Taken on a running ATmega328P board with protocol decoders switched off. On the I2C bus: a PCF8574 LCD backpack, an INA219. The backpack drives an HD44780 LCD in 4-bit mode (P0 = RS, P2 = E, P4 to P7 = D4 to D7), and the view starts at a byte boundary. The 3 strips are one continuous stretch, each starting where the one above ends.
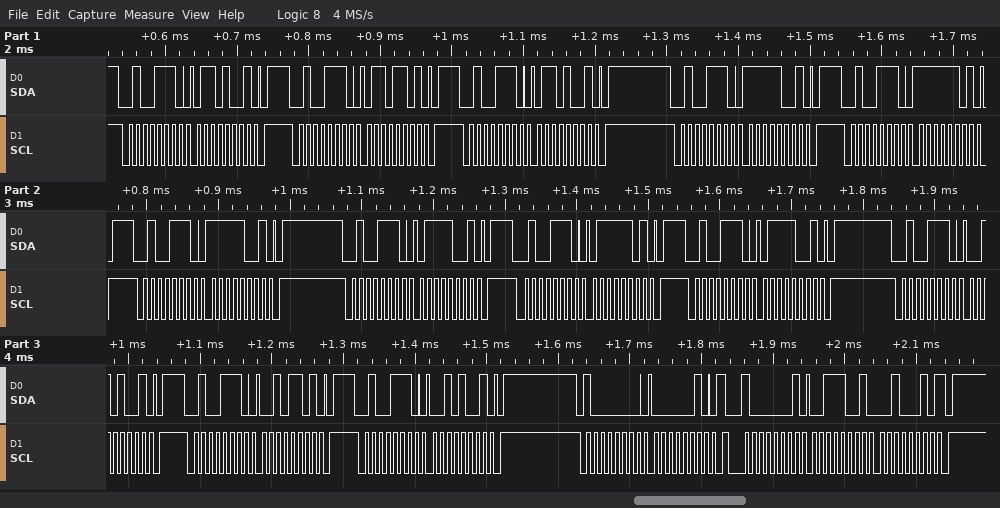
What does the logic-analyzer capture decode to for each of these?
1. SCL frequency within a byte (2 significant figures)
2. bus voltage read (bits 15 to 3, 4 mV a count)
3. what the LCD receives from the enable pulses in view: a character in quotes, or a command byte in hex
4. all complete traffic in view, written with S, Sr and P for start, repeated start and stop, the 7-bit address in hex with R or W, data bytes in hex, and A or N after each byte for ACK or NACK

100 kHz
7.312 V
'o' 'r'
S 27W A 69 A P S 27W A 6D A P S 27W A 69 A P S 27W A F9 A P S 27W A FD A P S 27W A F9 A P S 27W A 79 A P S 27W A 7D A P S 27W A 79 A P S 27W A 29 A P S 27W A 2D A P S 27W A 29 A P S 40W A 02 A Sr 40R A 39 A 22 N P
